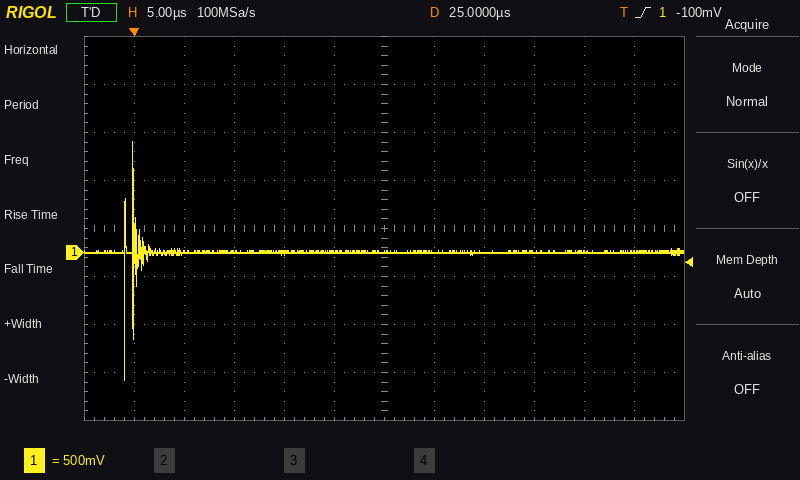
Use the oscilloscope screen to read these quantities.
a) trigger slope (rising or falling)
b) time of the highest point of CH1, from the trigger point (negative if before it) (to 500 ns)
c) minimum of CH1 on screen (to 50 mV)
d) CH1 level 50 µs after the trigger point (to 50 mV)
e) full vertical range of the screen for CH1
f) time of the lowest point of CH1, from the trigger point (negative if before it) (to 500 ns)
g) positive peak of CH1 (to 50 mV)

rising
0.0 µs
-1.30 V
0 mV
4 V
-1.0 µs
1.15 V
